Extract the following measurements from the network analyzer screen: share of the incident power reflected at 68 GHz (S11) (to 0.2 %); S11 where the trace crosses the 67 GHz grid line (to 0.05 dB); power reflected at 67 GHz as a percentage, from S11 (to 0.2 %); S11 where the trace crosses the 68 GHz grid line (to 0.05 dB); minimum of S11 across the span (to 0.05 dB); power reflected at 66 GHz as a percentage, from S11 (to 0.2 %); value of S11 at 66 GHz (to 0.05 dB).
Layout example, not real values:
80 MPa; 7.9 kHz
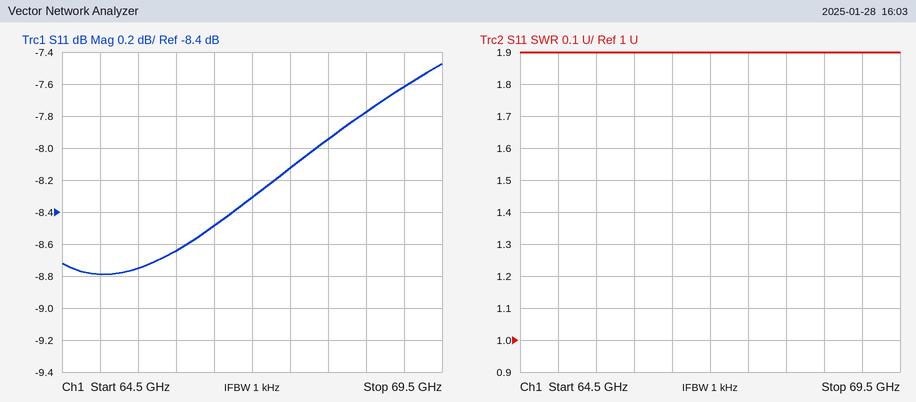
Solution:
16.0 %; -8.30 dB; 14.8 %; -7.95 dB; -8.80 dB; 13.6 %; -8.65 dB
